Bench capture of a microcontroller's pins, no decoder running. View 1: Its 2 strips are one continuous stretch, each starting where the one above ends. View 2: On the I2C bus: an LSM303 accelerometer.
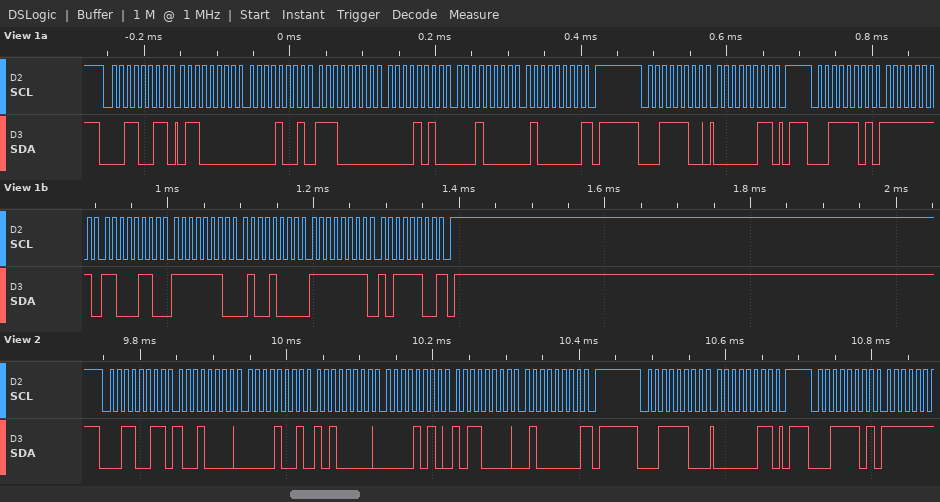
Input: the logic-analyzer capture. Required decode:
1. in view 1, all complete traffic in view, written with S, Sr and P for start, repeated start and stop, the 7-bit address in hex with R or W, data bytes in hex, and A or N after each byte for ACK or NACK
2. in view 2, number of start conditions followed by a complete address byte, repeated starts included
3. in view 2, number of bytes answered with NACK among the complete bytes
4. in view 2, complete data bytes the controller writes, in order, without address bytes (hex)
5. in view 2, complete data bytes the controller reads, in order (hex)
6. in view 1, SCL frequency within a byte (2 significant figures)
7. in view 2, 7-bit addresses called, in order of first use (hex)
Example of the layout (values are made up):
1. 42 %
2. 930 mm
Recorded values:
1. S 19R A 60 A 09 A E0 A 0A A 10 A 40 N P S 1EW A 03 A P S 1ER A FF A C6 A FE A 48 A FF A BC N P
2. 3
3. 1
4. 03
5. 90 09 A0 0A B0 40
6. 100 kHz
7. 0x19 0x1E
